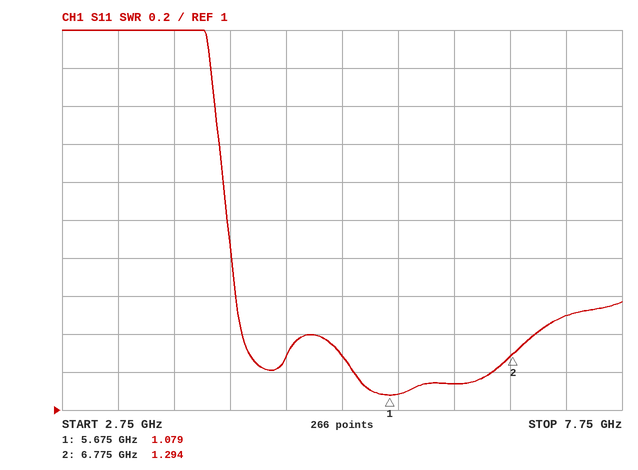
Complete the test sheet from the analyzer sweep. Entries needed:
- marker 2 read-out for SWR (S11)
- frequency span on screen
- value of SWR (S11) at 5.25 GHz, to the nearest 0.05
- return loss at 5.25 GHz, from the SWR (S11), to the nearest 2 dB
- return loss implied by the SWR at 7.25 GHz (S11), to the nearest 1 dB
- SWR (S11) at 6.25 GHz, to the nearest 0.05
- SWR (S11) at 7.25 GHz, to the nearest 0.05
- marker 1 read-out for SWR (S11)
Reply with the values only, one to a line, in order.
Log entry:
1.294
5 GHz
1.30
18 dB
14 dB
1.15
1.50
1.079
